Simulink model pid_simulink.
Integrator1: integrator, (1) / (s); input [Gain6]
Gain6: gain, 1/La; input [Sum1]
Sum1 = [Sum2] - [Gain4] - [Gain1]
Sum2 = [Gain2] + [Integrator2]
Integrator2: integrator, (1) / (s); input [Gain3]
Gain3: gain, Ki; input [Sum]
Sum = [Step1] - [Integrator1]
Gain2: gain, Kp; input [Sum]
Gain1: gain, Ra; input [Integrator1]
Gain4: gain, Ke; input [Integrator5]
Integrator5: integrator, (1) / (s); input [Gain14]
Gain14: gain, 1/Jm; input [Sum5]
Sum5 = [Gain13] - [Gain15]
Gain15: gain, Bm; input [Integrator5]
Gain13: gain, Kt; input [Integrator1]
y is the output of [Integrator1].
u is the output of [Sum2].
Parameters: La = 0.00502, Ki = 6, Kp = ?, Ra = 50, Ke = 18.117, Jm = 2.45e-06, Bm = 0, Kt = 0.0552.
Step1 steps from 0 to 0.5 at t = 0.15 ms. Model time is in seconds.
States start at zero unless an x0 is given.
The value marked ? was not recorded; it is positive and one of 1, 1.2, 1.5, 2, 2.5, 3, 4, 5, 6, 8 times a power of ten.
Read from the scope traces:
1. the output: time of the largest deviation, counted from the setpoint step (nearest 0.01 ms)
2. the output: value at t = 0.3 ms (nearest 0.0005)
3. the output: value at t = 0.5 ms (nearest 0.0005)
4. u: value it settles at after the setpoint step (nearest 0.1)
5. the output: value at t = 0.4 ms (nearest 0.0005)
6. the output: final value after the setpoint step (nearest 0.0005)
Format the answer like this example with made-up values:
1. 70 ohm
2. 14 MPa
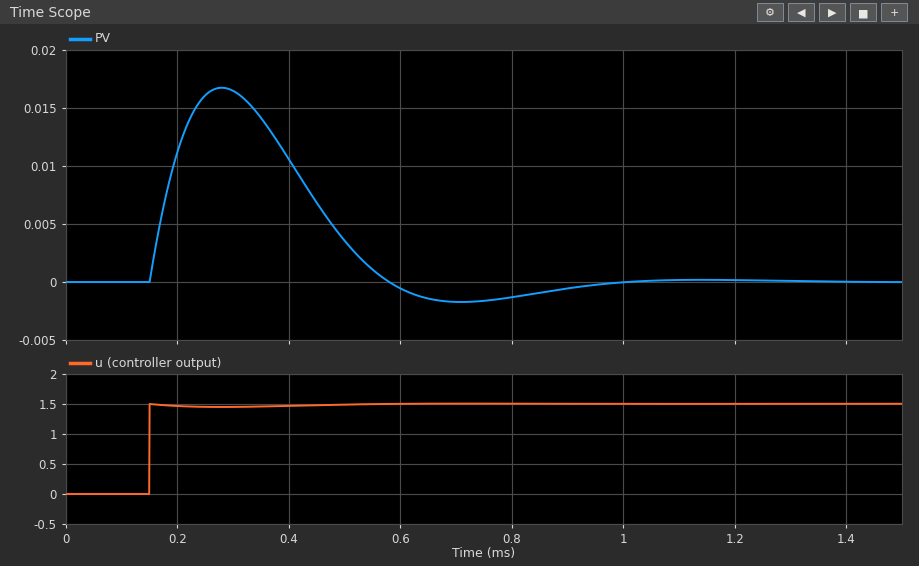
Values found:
1. 0.13 ms
2. 0.0165
3. 0.0035
4. 1.5
5. 0.0105
6. 0.0000
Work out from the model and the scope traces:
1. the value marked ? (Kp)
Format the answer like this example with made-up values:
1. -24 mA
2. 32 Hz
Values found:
1. 3
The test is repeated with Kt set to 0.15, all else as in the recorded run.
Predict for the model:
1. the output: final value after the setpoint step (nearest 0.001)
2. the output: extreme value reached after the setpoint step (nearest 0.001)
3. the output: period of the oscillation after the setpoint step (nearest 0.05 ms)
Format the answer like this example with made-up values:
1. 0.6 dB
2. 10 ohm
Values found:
1. 0.000
2. 0.013
3. 0.45 ms
